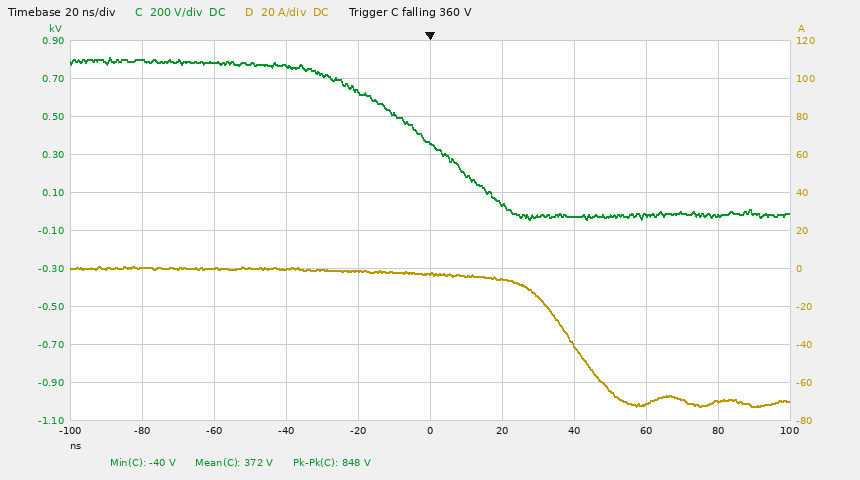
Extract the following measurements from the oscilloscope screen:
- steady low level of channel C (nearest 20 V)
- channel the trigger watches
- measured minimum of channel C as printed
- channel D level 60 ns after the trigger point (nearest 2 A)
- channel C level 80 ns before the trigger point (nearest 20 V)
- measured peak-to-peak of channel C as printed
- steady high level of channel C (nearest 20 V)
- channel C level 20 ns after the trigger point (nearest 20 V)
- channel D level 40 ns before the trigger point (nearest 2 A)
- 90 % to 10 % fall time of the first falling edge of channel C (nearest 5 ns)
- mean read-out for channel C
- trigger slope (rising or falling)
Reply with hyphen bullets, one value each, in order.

- -20 V
- channel C
- -40 V
- -72 A
- 800 V
- 848 V
- 780 V
- 40 V
- 0 A
- 45 ns
- 372 V
- falling
